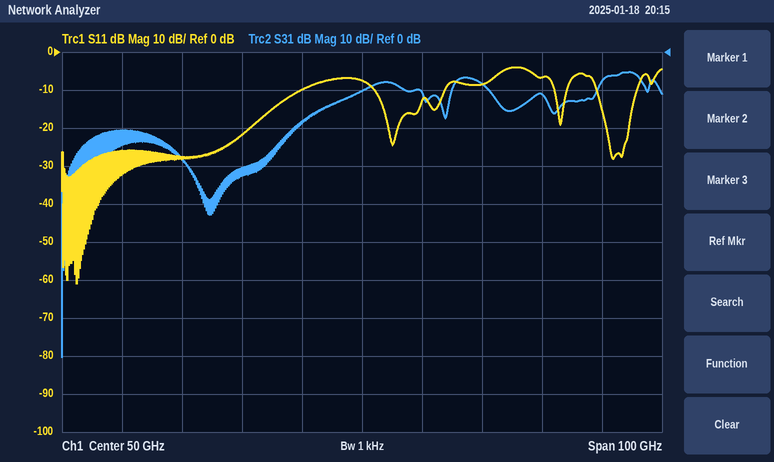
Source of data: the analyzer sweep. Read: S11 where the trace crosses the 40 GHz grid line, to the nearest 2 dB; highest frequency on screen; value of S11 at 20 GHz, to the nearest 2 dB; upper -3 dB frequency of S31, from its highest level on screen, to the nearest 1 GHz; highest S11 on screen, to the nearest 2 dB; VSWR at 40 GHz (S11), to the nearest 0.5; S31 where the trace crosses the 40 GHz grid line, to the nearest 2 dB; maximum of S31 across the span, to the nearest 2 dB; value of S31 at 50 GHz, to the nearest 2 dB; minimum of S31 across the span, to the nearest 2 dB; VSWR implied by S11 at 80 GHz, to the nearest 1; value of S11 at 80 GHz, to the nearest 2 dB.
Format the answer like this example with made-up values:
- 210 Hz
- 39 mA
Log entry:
- -10 dB
- 100 GHz
- -28 dB
- 97 GHz
- -4 dB
- 2.0
- -18 dB
- -6 dB
- -10 dB
- -80 dB
- 3
- -6 dB
